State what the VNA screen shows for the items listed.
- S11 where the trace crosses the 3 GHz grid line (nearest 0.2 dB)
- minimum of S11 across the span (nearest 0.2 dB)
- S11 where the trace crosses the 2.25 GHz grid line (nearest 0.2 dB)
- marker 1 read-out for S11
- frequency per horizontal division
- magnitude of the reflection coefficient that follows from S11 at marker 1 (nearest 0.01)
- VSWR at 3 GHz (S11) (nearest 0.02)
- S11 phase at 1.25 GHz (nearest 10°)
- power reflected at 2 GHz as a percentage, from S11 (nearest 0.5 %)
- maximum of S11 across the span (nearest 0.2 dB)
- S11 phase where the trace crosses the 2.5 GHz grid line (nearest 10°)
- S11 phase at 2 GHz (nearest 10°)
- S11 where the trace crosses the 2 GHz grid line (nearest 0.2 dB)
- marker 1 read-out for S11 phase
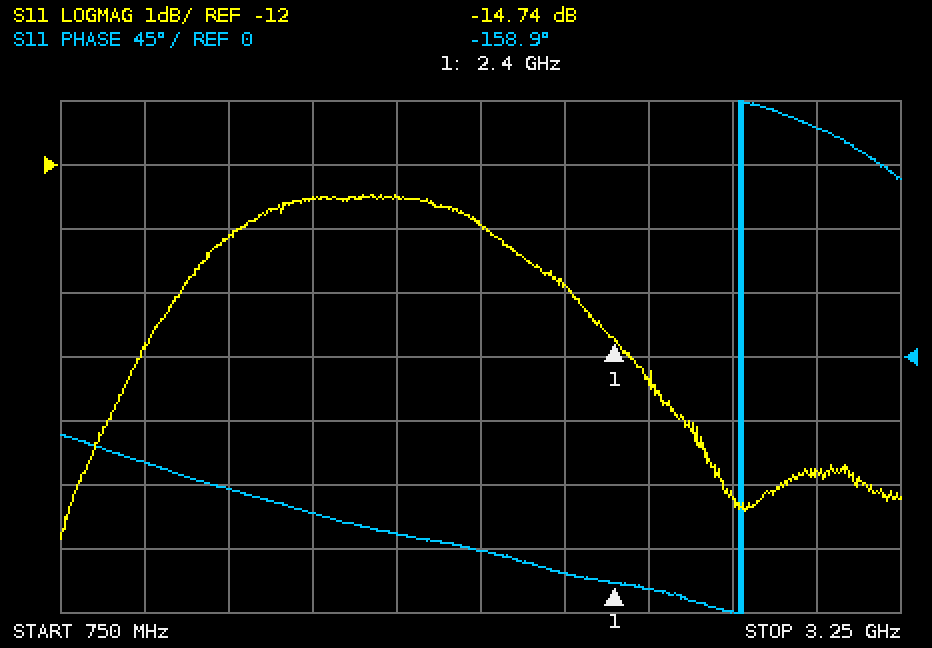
-16.8 dB
-17.8 dB
-13.8 dB
-14.74 dB
250 MHz
0.18
1.34
-90°
5.0 %
-12.4 dB
-160°
-140°
-13.0 dB
-158.9°
